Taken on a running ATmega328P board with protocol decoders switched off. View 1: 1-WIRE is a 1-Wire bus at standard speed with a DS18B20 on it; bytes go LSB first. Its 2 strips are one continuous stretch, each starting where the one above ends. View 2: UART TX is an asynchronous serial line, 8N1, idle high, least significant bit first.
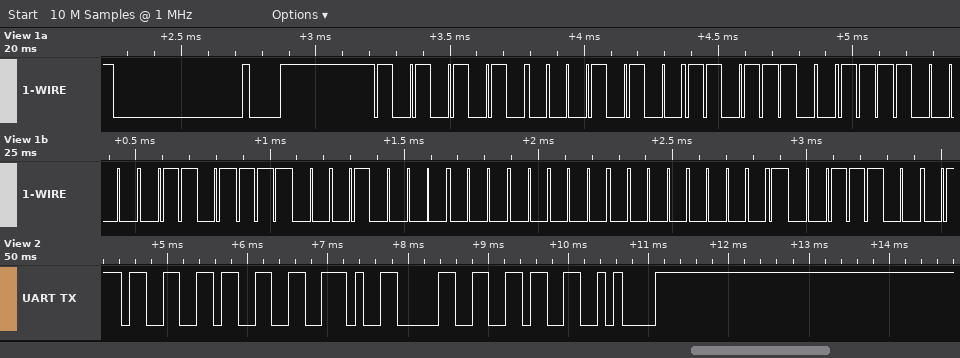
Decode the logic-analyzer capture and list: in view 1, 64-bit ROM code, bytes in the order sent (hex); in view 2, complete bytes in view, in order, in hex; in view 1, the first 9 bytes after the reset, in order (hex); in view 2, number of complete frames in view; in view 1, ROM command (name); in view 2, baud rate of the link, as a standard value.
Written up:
28 3B 0F F6 08 00 00 39
33 33 2E 30 36 0A
55 28 3B 0F F6 08 00 00 39
6
Match ROM
9600 baud
